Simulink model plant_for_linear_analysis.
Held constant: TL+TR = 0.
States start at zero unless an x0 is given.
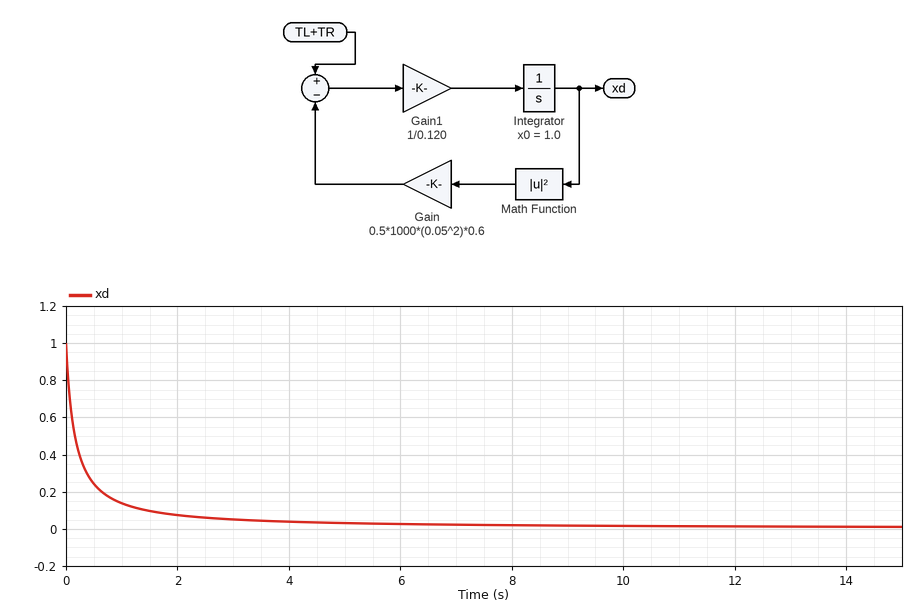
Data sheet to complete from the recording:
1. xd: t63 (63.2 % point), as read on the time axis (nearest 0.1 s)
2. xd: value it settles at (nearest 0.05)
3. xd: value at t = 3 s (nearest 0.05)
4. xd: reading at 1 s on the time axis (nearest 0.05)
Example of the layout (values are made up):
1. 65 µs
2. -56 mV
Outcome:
1. 0.3 s
2. 0.00
3. 0.05
4. 0.15
